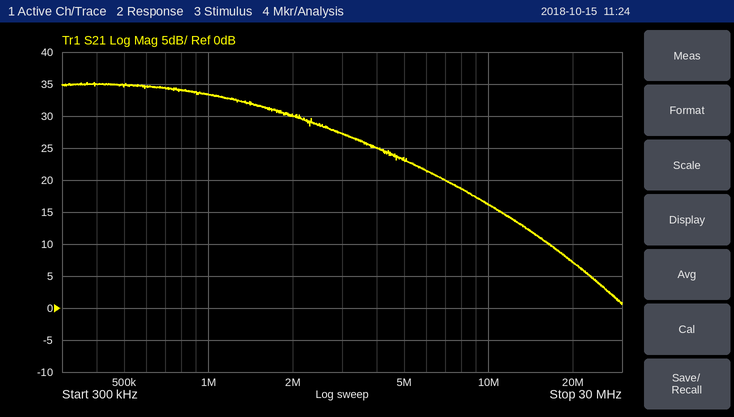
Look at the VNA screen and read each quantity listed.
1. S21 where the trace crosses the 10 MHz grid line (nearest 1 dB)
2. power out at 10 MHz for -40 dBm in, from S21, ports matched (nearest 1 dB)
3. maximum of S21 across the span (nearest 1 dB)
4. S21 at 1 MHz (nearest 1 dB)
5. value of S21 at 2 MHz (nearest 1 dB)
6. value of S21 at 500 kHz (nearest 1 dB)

16 dB
-24 dBm
35 dB
33 dB
30 dB
35 dB
